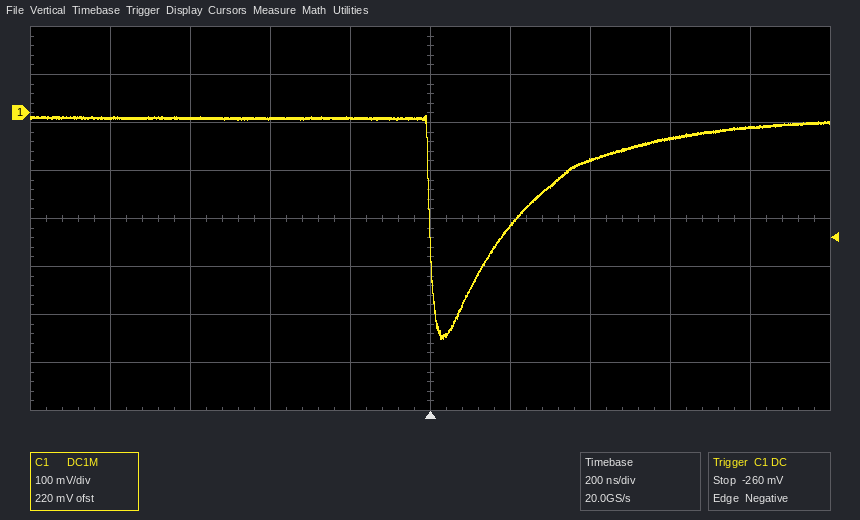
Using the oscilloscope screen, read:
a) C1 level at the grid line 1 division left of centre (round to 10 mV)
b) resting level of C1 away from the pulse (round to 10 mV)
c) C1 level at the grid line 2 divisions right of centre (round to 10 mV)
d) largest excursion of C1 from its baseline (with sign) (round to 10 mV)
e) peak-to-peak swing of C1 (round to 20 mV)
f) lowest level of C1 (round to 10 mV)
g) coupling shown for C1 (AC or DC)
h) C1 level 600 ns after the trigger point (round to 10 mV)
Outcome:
-10 mV
-10 mV
-100 mV
-460 mV
460 mV
-470 mV
DC
-50 mV
